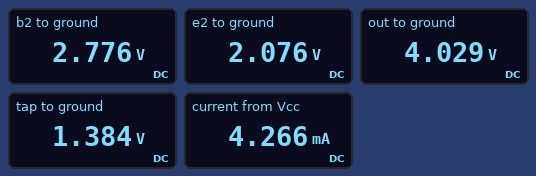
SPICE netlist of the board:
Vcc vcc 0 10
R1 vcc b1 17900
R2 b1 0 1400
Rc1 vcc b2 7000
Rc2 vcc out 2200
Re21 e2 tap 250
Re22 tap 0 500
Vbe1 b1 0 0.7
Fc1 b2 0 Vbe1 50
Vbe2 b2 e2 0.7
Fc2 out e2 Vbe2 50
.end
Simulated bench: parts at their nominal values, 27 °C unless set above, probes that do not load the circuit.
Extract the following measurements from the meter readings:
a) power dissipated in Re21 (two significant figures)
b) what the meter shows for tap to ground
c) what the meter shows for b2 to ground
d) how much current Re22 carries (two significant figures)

1.9 mW
1.384 V
2.776 V
2.8 mA
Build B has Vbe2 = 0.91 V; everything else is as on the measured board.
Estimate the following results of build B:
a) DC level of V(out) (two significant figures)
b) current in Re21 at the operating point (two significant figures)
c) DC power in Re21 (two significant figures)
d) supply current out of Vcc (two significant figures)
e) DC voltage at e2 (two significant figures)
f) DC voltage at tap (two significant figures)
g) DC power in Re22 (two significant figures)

4.5 V
2.5 mA
1.6 mW
4.0 mA
1.9 V
1.3 V
3.2 mW
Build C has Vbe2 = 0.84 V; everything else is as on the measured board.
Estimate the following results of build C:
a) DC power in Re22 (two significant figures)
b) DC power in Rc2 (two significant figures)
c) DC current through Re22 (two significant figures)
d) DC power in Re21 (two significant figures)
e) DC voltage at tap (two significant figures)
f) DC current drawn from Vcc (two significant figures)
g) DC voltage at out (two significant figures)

3.4 mW
14 mW
2.6 mA
1.7 mW
1.3 V
4.1 mA
4.4 V
